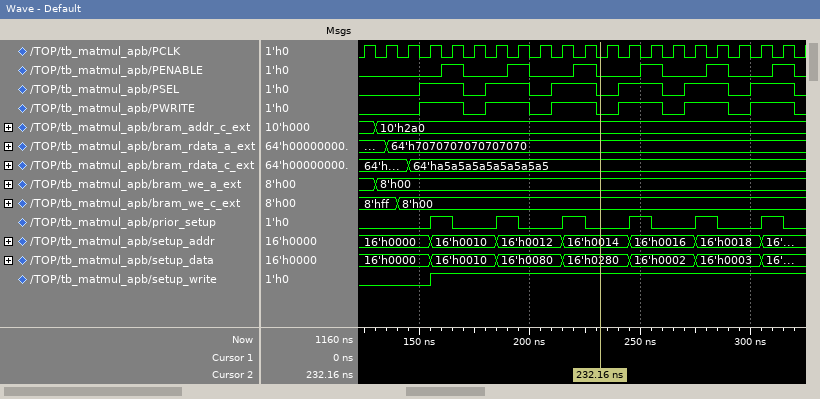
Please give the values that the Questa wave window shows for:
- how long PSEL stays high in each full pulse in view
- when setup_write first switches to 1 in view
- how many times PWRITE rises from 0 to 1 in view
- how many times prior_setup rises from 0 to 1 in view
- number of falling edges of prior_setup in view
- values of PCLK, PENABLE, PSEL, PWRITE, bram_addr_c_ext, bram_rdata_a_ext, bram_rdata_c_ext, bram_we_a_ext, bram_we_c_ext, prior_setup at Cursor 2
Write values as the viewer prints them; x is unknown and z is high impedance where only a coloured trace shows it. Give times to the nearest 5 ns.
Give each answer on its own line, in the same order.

20 ns, 20 ns, 20 ns, 20 ns, 20 ns, 20 ns
155 ns
6
6
6
PCLK=0, PENABLE=0, PSEL=0, PWRITE=0, bram_addr_c_ext=10'h2a0, bram_rdata_a_ext=64'h7070707070707070, bram_rdata_c_ext=64'ha5a5a5a5a5a5a5a5, bram_we_a_ext=8'h00, bram_we_c_ext=8'h00, prior_setup=0
